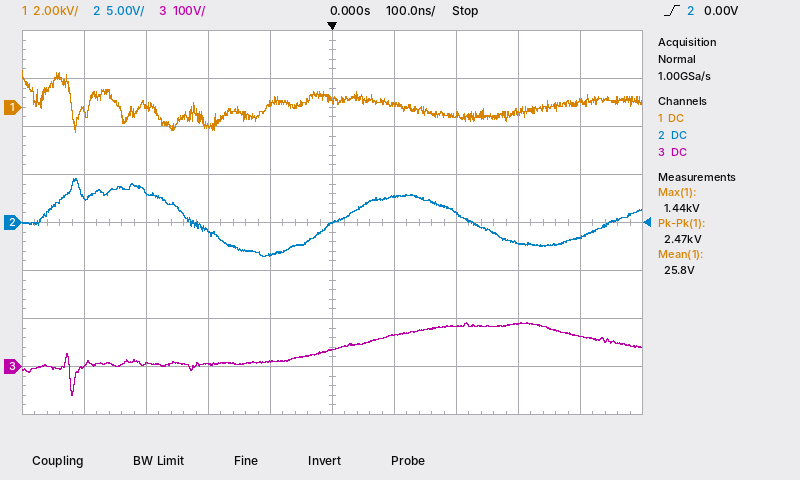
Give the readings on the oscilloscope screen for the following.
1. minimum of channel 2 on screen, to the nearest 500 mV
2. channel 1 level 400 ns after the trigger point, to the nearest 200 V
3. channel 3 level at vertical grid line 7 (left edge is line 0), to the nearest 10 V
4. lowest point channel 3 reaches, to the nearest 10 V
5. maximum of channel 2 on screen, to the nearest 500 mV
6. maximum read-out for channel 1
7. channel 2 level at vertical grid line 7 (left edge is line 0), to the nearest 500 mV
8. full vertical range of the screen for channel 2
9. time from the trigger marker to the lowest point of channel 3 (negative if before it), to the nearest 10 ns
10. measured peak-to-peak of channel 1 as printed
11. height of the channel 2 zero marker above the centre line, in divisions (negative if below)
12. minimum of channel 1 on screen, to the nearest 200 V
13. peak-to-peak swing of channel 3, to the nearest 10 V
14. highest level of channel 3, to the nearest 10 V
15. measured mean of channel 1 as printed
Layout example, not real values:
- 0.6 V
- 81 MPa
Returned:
- -3.5 V
- 200 V
- 80 V
- -60 V
- 4.5 V
- 1.44 kV
- 1.0 V
- 40 V
- -420 ns
- 2.47 kV
- 0.0 div
- -1.0 kV
- 150 V
- 90 V
- 25.8 V
